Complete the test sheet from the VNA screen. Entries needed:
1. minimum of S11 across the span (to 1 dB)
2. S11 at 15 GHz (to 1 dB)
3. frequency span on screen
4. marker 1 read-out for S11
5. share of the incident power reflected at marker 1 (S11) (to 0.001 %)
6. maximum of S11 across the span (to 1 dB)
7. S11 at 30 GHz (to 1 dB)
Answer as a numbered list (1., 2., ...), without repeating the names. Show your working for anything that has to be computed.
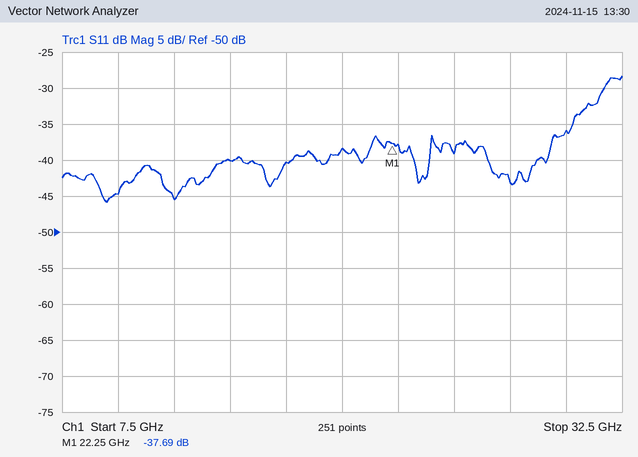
1. -46 dB
2. -40 dB
3. 25 GHz
4. -37.69 dB
5. 10^(-37.69/10) ≈ 0.017 %
6. -28 dB
7. -36 dB
